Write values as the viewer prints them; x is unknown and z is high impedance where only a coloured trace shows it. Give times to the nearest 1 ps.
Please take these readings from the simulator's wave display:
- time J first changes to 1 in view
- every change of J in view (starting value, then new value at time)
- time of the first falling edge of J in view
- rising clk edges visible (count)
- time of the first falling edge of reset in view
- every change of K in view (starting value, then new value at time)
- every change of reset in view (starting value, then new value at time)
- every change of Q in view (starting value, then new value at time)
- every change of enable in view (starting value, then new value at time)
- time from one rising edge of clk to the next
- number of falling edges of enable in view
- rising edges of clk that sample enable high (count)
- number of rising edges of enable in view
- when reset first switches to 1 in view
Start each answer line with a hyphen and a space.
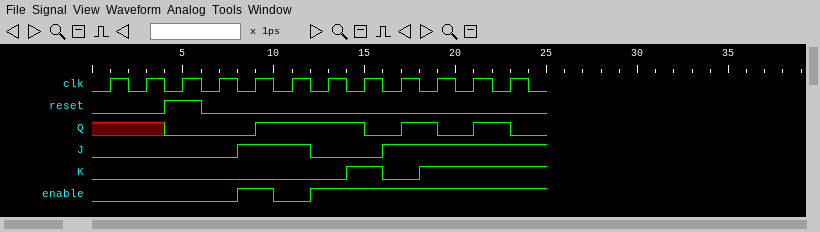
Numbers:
- 8 ps
- 0, 1 at 8 ps, 0 at 12 ps, 1 at 16 ps
- 12 ps
- 12
- 6 ps
- 0, 1 at 14 ps, 0 at 16 ps, 1 at 18 ps
- 0, 1 at 4 ps, 0 at 6 ps
- x, 0 at 4 ps, 1 at 9 ps, 0 at 15 ps, 1 at 17 ps, 0 at 19 ps, 1 at 21 ps, 0 at 23 ps
- 0, 1 at 8 ps, 0 at 10 ps, 1 at 12 ps
- 2 ps
- 1
- 7
- 2
- 4 ps
